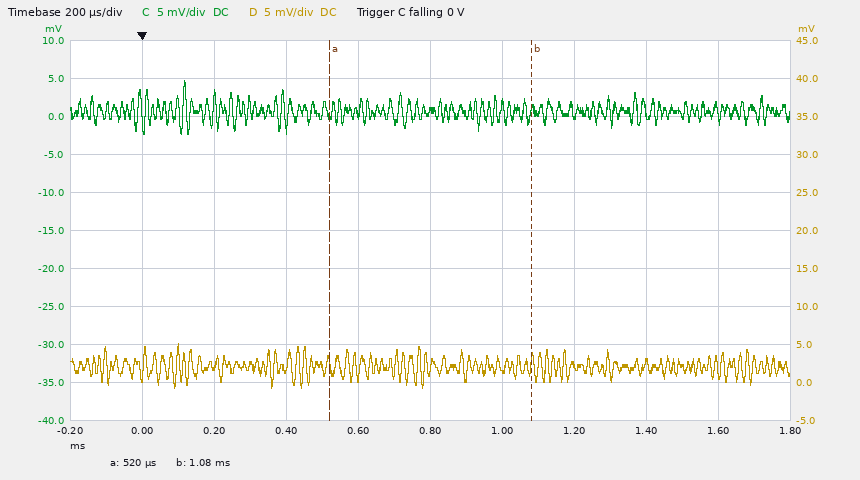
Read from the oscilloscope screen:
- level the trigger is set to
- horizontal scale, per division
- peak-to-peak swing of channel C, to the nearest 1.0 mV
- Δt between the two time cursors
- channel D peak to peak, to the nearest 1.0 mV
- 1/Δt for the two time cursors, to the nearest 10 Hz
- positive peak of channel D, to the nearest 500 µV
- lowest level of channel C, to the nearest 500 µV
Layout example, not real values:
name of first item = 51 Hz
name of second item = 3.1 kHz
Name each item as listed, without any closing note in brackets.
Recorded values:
level the trigger is set to = 0 V
horizontal scale, per division = 200 µs
peak-to-peak swing of channel C, to the nearest 1.0 mV = 7.0 mV
Δt between the two time cursors = 560 µs
channel D peak to peak, to the nearest 1.0 mV = 6.0 mV
1/Δt for the two time cursors, to the nearest 10 Hz = 1.79 kHz
positive peak of channel D, to the nearest 500 µV = 5.0 mV
lowest level of channel C, to the nearest 500 µV = -2.5 mV
